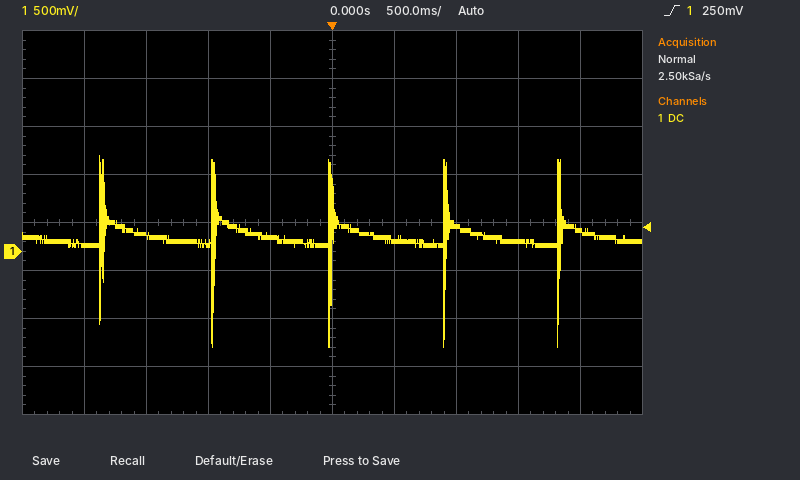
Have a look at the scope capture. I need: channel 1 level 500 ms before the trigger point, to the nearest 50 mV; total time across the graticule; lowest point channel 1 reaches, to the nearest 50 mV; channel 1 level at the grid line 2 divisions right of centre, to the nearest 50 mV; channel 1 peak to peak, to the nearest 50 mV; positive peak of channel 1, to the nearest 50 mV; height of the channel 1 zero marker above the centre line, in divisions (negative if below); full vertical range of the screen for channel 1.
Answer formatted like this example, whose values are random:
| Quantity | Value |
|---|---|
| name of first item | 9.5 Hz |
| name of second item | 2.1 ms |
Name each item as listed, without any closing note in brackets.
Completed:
| Quantity | Value |
|---|---|
| channel 1 level 500 ms before the trigger point, to the nearest 50 mV | 150 mV |
| total time across the graticule | 5 s |
| lowest point channel 1 reaches, to the nearest 50 mV | -1.00 V |
| channel 1 level at the grid line 2 divisions right of centre, to the nearest 50 mV | 300 mV |
| channel 1 peak to peak, to the nearest 50 mV | 2.00 V |
| positive peak of channel 1, to the nearest 50 mV | 1.00 V |
| height of the channel 1 zero marker above the centre line, in divisions | -0.6 div |
| full vertical range of the screen for channel 1 | 4 V |
